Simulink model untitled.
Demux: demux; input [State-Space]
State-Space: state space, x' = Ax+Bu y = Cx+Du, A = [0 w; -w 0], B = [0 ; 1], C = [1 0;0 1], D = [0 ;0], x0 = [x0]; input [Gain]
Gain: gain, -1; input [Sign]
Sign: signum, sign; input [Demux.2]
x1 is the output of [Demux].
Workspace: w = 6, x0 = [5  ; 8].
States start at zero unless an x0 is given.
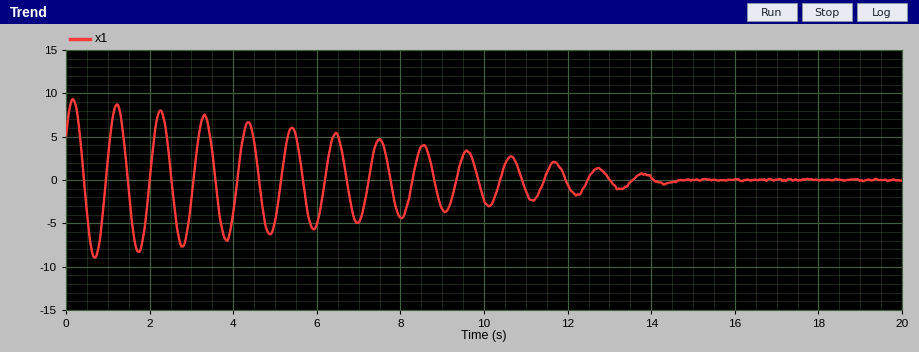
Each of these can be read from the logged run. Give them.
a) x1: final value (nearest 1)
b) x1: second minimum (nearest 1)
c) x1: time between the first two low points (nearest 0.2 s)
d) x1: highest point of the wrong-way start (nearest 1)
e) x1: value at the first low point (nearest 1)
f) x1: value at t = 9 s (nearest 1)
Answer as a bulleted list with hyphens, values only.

- 0
- -8
- 1.0 s
- 9
- -9
- -3
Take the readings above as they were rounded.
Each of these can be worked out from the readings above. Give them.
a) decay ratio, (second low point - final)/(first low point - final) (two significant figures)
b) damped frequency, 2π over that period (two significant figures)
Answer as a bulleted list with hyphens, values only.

- 0.89
- 6.3 rad/s
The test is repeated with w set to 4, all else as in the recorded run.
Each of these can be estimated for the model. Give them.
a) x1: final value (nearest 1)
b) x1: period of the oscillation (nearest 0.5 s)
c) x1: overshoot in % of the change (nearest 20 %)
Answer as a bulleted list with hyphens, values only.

- 0
- 1.5 s
- 180 %
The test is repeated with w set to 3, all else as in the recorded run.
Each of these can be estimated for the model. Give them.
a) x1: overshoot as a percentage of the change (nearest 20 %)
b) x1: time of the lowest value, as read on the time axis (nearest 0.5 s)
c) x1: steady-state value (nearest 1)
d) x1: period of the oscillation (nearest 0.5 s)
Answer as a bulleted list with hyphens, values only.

- 180 %
- 1.5 s
- 0
- 2.0 s
